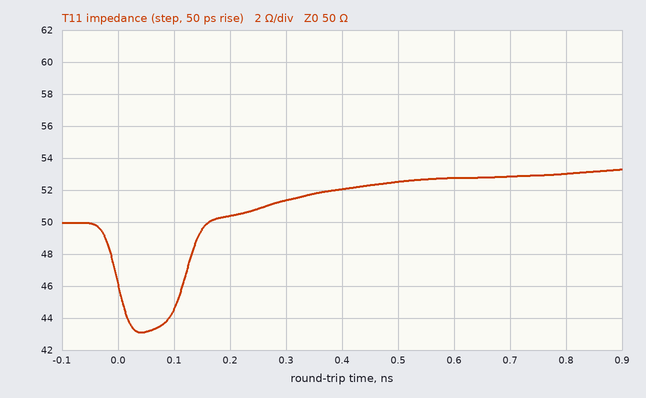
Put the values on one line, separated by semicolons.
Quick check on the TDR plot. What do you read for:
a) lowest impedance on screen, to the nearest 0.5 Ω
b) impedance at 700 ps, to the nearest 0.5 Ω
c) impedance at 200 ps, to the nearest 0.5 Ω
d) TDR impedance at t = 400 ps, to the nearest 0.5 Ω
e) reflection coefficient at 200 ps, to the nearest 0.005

43.0 Ω; 53.0 Ω; 50.5 Ω; 52.0 Ω; +0.005
